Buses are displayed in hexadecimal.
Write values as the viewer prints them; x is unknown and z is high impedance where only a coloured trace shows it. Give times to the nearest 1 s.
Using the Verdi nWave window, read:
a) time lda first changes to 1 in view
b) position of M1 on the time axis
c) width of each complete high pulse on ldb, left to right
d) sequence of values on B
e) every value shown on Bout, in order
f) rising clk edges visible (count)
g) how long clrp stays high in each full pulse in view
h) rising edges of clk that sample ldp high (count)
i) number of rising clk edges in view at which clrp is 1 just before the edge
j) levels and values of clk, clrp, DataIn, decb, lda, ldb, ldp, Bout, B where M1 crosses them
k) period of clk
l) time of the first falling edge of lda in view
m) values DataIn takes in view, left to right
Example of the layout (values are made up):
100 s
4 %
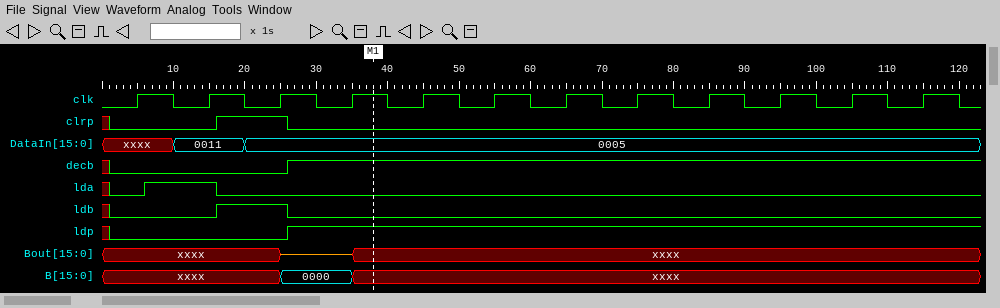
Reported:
6 s
38 s
10 s
xxxx, 0000, xxxx
xxxx, z, xxxx
12
10 s
9
1
clk=1, clrp=0, DataIn=0005, decb=1, lda=0, ldb=0, ldp=1, Bout=xxxx, B=xxxx
10 s
16 s
xxxx, 0011, 0005
